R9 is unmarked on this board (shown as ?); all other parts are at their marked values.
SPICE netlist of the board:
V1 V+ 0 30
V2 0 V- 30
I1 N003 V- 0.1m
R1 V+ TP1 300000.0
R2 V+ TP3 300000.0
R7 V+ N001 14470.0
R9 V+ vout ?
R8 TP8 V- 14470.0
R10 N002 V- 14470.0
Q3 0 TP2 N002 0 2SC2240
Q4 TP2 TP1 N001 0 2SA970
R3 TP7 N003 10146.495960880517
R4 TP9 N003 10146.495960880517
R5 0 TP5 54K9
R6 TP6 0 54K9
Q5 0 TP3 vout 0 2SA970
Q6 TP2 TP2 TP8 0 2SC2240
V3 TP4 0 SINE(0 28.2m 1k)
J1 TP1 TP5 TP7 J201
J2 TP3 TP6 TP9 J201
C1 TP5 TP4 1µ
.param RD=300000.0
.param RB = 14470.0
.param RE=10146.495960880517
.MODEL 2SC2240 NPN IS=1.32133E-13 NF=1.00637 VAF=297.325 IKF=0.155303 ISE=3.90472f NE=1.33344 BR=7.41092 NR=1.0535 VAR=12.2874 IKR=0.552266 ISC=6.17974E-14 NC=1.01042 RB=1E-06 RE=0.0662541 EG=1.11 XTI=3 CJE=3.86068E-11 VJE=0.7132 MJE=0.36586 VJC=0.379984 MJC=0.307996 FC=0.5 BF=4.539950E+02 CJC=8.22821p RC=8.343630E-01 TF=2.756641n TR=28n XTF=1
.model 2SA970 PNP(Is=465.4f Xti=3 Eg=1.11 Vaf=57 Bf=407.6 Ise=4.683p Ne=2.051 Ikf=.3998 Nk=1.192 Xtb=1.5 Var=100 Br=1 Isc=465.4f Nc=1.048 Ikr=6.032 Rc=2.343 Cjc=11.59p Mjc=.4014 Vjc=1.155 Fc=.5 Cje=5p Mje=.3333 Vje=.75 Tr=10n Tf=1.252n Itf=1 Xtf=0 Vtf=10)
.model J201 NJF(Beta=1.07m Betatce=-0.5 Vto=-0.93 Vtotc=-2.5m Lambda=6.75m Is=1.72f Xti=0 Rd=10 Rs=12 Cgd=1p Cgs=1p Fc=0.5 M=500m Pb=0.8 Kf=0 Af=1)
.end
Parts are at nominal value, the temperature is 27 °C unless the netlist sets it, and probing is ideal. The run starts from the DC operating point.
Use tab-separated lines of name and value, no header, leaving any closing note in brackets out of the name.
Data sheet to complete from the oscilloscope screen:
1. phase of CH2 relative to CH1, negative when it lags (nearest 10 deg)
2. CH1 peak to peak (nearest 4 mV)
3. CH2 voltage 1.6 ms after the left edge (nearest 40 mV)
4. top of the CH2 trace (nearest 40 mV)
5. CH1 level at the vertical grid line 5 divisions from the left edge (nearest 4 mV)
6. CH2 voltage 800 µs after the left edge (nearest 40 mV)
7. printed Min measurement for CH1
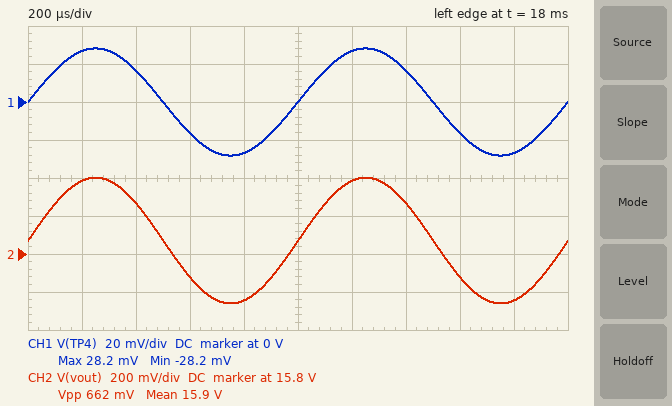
phase of CH2 relative to CH1, negative when it lags	0 deg
CH1 peak to peak	56 mV
CH2 voltage 1.6 ms after the left edge	15.68 V
top of the CH2 trace	16.20 V
CH1 level at the vertical grid line 5 divisions from the left edge	0 V
CH2 voltage 800 µs after the left edge	15.56 V
printed Min measurement for CH1	-28.2 mV
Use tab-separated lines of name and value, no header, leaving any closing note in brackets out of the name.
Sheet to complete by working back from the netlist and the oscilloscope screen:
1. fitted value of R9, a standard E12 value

fitted value of R9, a standard E12 value	27 kΩ
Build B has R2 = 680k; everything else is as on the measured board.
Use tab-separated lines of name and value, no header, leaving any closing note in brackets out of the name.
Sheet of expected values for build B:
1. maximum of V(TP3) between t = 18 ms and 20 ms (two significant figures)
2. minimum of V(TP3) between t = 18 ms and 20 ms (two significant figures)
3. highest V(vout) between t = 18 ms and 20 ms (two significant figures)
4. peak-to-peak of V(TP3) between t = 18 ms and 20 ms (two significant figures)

maximum of V(TP3) between t = 18 ms and 20 ms	750 mV
minimum of V(TP3) between t = 18 ms and 20 ms	680 mV
highest V(vout) between t = 18 ms and 20 ms	1.3 V
peak-to-peak of V(TP3) between t = 18 ms and 20 ms	74 mV
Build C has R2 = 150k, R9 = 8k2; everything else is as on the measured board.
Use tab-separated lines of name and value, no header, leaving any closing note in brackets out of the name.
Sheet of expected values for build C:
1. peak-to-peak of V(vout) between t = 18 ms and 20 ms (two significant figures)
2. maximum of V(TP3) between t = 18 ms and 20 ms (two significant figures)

peak-to-peak of V(vout) between t = 18 ms and 20 ms	330 mV
maximum of V(TP3) between t = 18 ms and 20 ms	23 V
